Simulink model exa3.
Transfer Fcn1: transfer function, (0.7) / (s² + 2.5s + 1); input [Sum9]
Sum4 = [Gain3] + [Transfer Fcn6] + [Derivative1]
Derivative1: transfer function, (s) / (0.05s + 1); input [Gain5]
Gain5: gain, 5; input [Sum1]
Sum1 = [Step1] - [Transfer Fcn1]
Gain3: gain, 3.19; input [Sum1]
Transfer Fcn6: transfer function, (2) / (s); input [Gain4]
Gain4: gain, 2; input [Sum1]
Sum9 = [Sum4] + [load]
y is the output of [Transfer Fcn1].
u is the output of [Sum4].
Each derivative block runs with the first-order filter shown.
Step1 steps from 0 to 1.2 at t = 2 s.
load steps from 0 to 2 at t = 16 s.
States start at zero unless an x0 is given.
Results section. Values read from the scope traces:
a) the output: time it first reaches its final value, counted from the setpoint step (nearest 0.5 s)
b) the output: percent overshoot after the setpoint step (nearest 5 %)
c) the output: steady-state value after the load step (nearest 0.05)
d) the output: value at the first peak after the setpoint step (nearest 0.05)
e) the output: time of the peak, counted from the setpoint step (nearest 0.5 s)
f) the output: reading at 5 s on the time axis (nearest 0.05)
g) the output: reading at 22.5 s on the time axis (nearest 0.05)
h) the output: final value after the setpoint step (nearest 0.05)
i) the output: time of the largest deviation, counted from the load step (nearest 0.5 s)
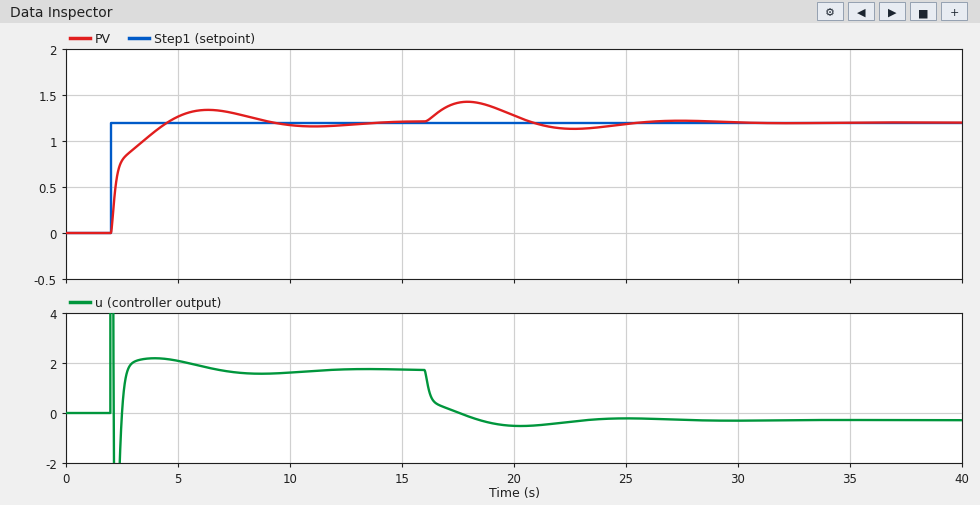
2.5 s
10 %
1.20
1.35
4.5 s
1.25
1.15
1.20
2.0 s
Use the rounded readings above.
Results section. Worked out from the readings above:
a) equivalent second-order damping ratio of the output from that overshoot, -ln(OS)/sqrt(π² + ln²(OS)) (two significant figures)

0.59
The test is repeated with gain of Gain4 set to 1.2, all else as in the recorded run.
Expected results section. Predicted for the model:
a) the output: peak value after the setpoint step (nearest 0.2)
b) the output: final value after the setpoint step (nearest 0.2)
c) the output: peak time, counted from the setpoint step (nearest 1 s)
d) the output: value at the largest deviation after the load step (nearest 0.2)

1.2
1.2
6 s
1.4
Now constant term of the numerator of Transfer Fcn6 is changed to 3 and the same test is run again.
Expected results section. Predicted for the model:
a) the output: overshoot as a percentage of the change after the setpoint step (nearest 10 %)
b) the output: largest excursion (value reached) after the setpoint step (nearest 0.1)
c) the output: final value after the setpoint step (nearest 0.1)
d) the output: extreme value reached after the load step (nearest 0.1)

20 %
1.4
1.2
1.4
